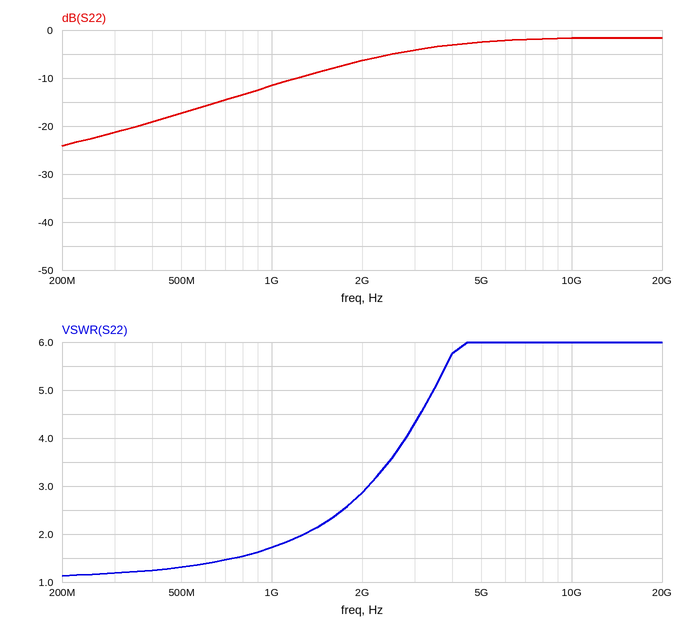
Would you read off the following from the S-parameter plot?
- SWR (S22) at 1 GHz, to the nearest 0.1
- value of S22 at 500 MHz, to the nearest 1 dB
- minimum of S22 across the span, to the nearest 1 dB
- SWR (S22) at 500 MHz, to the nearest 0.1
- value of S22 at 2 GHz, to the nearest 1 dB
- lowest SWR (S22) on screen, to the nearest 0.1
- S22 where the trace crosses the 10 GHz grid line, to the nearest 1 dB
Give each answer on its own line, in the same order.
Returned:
1.7
-17 dB
-24 dB
1.3
-6 dB
1.1
-2 dB
